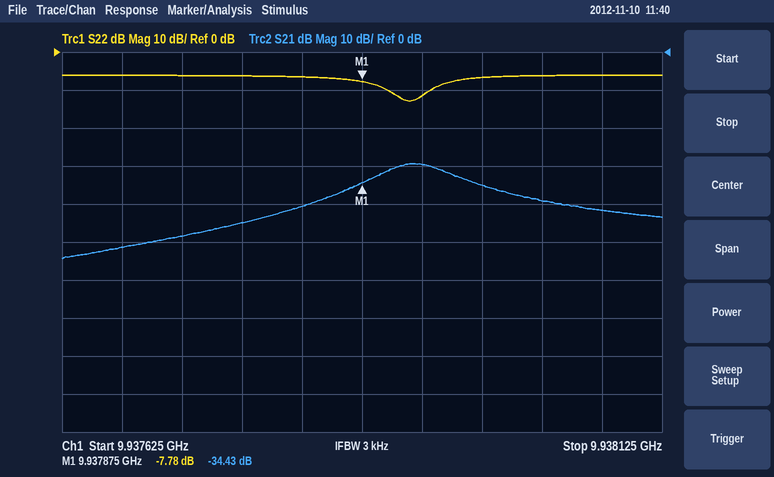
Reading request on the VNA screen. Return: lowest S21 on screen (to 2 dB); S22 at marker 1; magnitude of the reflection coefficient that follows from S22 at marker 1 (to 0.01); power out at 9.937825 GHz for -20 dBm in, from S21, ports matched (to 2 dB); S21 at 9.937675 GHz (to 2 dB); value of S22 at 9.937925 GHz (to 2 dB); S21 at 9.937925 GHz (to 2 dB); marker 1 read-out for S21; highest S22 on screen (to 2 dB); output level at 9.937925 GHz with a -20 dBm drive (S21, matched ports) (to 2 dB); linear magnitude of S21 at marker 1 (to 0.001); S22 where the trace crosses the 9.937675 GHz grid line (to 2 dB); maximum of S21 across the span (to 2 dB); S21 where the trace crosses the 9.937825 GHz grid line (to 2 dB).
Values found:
-54 dB
-7.78 dB
0.41
-60 dBm
-52 dB
-12 dB
-30 dB
-34.43 dB
-6 dB
-50 dBm
0.019
-6 dB
-30 dB
-40 dB
